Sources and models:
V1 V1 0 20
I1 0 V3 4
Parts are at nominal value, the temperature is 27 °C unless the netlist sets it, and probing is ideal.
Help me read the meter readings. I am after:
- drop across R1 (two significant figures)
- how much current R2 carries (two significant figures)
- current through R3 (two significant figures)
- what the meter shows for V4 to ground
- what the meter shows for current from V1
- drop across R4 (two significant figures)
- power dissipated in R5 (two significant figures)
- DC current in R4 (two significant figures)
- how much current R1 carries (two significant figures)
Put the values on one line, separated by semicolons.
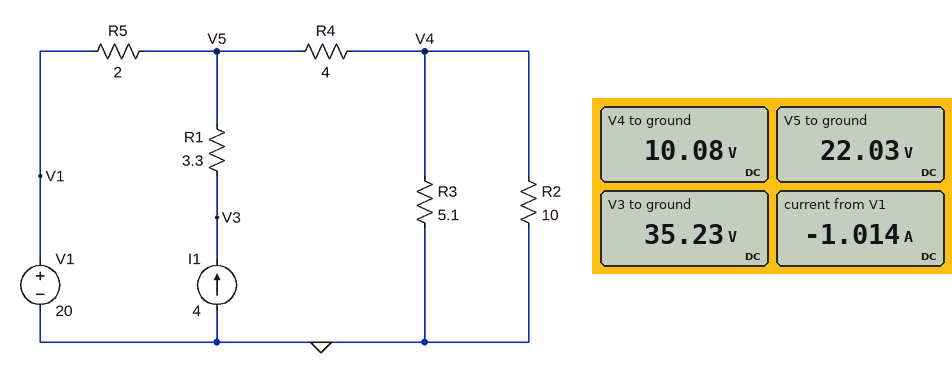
13 V; 1.0 A; 2.0 A; 10.08 V; -1.014 A; 12 V; 2.1 W; 3.0 A; 4.0 A
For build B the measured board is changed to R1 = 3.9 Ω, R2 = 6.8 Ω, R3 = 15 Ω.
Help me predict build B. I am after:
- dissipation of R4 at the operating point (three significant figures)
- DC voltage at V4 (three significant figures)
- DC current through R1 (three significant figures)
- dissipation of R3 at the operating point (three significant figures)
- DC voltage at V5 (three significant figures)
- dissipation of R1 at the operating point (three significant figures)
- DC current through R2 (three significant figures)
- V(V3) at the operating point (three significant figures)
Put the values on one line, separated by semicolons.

27.5 W; 12.3 V; 4.00 A; 10.0 W; 22.8 V; 62.4 W; 1.80 A; 38.4 V
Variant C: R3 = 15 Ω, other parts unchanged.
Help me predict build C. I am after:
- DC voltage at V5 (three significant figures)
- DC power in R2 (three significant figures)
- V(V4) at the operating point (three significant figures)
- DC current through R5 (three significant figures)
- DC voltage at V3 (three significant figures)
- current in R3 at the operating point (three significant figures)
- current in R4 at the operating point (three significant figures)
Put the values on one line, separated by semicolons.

23.3 V; 19.6 W; 14.0 V; 1.67 A; 36.5 V; 933 mA; 2.33 A
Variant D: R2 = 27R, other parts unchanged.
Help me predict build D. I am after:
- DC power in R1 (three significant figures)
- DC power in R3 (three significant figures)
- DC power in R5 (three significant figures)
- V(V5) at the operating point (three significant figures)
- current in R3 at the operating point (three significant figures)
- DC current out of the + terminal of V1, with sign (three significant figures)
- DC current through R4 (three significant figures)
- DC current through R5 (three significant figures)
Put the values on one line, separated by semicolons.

52.8 W; 26.7 W; 3.27 W; 22.6 V; 2.29 A; -1.28 A; 2.72 A; 1.28 A
